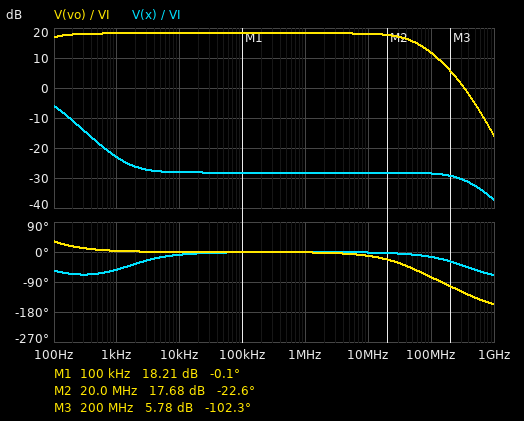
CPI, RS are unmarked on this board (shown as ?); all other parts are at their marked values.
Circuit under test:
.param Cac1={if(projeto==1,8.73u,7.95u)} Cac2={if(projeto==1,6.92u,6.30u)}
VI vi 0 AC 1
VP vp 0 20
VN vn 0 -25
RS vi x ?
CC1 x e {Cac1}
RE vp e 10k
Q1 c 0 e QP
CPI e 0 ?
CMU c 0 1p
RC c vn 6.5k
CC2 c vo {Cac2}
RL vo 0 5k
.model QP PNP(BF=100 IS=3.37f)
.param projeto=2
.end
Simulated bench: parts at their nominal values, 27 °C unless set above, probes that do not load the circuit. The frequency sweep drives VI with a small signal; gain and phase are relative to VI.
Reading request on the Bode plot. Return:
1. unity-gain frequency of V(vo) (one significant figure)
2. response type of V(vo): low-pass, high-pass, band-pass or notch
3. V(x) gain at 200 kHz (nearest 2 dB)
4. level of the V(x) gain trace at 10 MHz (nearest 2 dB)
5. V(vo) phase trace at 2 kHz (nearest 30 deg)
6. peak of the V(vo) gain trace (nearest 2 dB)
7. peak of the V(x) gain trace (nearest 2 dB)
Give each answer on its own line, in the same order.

300 MHz
low-pass
-28 dB
-28 dB
0 deg
18 dB
-6 dB
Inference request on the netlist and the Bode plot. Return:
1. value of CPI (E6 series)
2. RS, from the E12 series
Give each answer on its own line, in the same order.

33 pF
330 Ω
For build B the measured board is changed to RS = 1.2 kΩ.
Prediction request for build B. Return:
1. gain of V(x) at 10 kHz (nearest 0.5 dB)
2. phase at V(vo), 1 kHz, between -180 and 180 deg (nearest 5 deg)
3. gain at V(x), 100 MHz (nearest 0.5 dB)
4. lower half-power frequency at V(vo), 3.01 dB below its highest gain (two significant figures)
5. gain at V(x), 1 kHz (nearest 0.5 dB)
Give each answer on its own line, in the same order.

-39.0 dB
0 deg
-39.5 dB
17 Hz
-34.0 dB
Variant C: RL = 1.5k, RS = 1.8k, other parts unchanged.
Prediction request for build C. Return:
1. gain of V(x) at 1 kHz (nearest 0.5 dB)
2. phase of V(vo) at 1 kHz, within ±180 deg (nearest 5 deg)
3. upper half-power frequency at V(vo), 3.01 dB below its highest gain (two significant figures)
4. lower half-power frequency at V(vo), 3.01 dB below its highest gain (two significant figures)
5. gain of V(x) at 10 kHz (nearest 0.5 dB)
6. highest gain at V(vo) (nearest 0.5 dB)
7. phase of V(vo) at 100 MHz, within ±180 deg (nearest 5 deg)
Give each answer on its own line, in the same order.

-37.5 dB
0 deg
120 MHz
12 Hz
-42.5 dB
-3.5 dB
-55 deg
